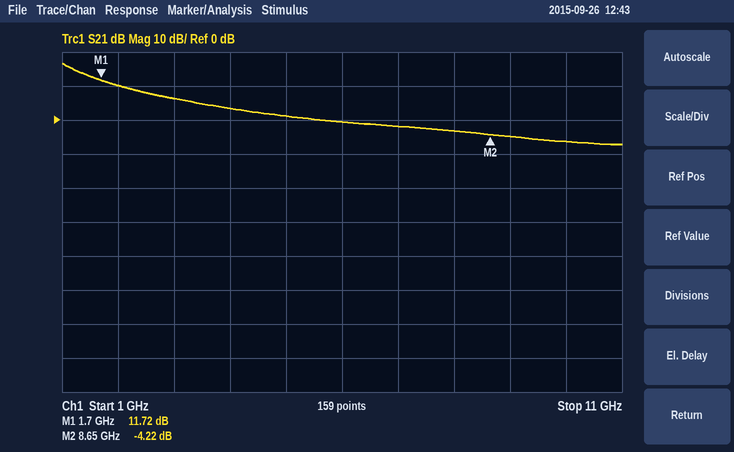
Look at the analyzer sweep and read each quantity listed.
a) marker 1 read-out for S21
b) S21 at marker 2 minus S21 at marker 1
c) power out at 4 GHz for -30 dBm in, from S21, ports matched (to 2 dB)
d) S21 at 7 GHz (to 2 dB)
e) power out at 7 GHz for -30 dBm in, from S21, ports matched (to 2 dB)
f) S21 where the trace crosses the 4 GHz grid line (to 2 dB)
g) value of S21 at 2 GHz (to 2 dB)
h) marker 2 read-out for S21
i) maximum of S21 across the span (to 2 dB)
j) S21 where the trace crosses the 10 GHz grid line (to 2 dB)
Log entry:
11.72 dB
-15.94 dB
-26 dBm
-2 dB
-32 dBm
4 dB
10 dB
-4.22 dB
16 dB
-6 dB
